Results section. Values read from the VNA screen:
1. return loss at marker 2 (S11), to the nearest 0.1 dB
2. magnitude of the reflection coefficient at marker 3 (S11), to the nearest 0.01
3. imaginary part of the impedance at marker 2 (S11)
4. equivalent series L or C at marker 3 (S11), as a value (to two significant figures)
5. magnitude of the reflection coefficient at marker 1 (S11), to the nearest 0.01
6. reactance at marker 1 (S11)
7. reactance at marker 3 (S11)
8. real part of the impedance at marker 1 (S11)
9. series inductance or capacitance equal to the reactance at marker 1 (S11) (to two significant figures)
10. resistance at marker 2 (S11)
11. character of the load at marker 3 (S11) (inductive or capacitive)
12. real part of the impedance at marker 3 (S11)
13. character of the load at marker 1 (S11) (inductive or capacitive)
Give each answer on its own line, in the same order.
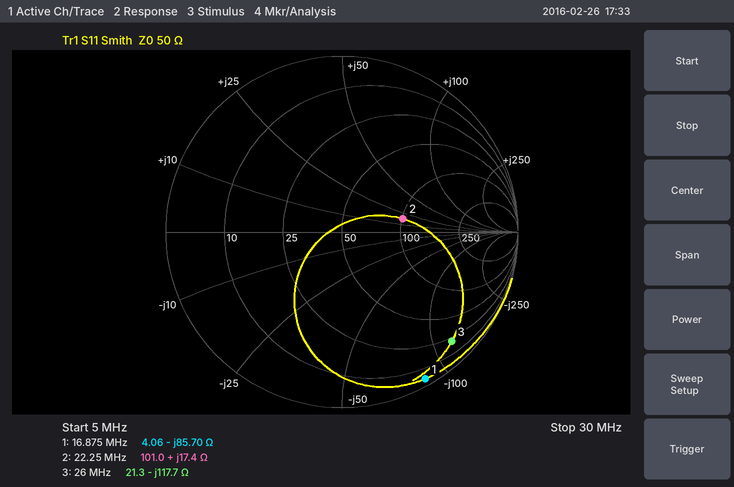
9.0 dB
0.88
+17.4 Ω
52 pF
0.96
-85.70 Ω
-117.7 Ω
4.06 Ω
110 pF
101.0 Ω
capacitive
21.3 Ω
capacitive
